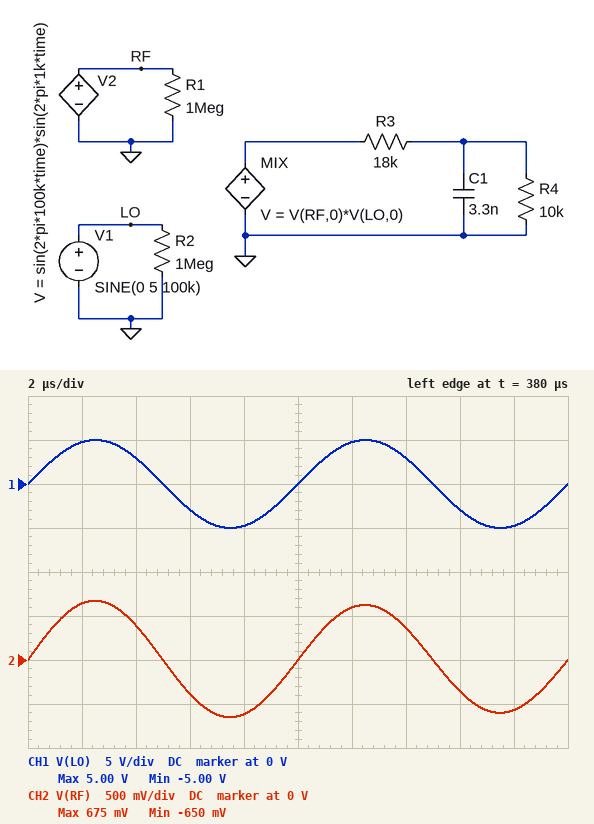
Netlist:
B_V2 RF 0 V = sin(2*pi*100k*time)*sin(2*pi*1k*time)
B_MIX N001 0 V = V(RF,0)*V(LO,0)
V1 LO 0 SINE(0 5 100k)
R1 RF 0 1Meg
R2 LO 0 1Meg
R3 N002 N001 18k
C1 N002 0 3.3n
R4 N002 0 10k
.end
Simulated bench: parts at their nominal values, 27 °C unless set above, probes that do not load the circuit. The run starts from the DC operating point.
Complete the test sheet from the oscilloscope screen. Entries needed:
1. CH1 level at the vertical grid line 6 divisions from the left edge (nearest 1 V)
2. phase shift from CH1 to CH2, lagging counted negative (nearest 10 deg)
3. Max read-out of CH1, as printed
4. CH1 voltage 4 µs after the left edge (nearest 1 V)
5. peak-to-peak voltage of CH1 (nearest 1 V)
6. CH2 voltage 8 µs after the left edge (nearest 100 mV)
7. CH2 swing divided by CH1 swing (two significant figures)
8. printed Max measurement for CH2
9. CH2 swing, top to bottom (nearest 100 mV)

5 V
0 deg
5.00 V
3 V
10 V
-600 mV
0.13
675 mV
1.3 V
